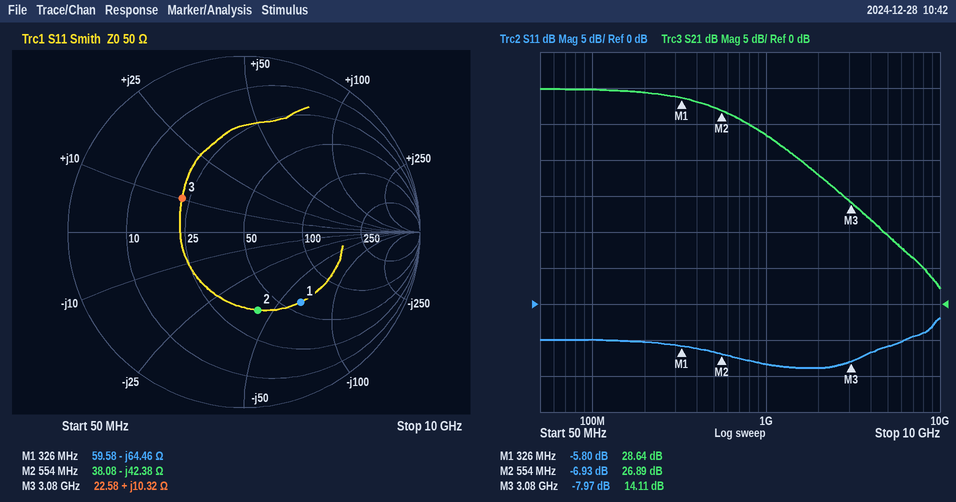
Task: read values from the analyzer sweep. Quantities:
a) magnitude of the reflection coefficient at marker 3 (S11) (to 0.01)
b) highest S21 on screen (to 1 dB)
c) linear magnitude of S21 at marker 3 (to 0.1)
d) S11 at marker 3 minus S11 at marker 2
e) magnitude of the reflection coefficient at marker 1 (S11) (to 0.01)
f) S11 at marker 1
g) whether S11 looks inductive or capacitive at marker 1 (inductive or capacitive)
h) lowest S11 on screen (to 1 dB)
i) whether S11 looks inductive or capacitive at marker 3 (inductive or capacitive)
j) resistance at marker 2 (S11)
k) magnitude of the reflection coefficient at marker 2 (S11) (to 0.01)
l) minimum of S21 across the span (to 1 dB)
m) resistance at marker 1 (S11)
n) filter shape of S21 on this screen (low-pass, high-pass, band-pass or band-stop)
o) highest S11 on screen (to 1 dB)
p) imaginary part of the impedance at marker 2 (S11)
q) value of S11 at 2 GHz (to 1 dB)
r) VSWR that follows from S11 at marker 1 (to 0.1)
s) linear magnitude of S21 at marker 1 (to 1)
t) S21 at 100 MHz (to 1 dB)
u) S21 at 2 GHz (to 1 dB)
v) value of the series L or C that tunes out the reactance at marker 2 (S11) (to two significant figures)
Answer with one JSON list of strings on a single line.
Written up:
["0.40", "30 dB", "5.1", "-1.04 dB", "0.51", "-5.80 dB", "capacitive", "-9 dB", "inductive", "38.08 Ω", "0.45", "2 dB", "59.58 Ω", "low-pass", "-2 dB", "-42.38 Ω", "-9 dB", "3.1", "27", "30 dB", "18 dB", "12 nH"]
